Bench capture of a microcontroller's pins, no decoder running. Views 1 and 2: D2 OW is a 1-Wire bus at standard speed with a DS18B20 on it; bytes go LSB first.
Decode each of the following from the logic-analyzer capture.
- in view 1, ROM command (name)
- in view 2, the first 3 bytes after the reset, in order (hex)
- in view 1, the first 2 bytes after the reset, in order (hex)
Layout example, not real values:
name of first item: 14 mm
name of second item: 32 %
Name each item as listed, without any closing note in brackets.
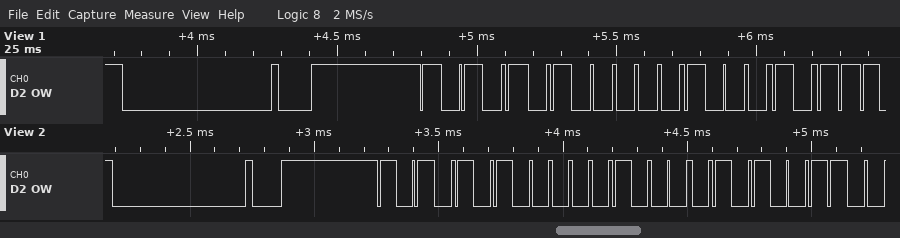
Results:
in view 1, ROM command: Match ROM
in view 2, the first 3 bytes after the reset, in order: 55 10 CA
in view 1, the first 2 bytes after the reset, in order: 55 10
